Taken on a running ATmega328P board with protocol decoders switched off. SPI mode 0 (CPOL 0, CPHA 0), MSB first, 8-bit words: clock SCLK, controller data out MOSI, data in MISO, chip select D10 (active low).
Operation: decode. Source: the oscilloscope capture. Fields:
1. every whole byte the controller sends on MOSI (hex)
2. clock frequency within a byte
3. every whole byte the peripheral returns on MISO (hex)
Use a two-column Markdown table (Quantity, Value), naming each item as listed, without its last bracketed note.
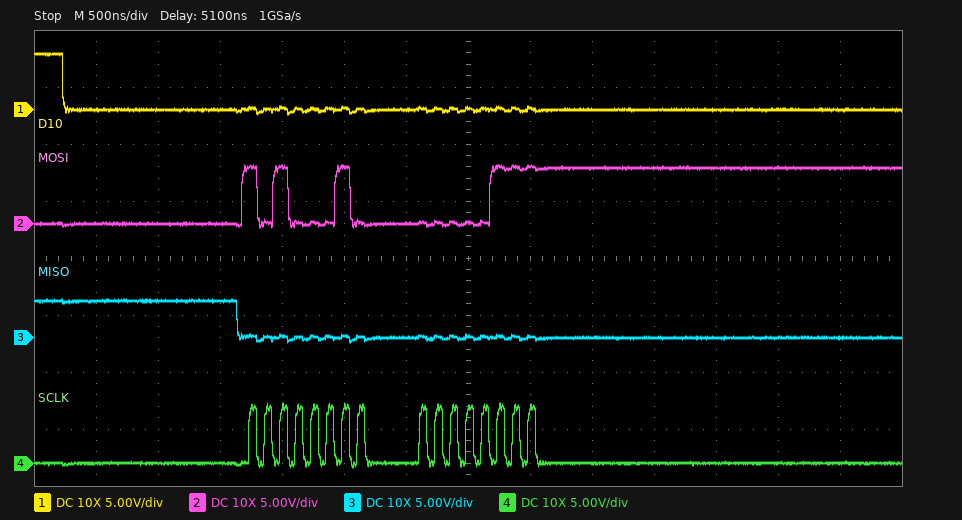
| Quantity | Value |
|---|---|
| every whole byte the controller sends on MOSI | A2 07 |
| clock frequency within a byte | 8 MHz |
| every whole byte the peripheral returns on MISO | 00 00 |
